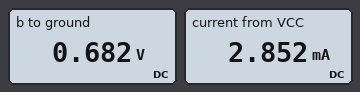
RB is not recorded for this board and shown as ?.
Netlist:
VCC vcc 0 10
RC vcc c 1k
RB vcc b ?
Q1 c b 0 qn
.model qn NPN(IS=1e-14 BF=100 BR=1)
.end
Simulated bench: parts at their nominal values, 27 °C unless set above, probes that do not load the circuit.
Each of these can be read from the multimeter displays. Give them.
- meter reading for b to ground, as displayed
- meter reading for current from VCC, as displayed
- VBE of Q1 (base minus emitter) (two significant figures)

0.682 V
2.852 mA
680 mV
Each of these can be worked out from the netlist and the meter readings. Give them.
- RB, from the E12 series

330 kΩ
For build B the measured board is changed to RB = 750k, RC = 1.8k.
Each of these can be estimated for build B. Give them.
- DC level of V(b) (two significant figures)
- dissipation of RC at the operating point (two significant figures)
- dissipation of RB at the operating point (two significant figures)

660 mV
2.8 mW
120 µW
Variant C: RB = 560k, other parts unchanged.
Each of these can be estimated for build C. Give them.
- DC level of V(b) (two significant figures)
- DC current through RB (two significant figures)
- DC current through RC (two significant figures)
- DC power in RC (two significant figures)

670 mV
17 µA
1.7 mA
2.8 mW
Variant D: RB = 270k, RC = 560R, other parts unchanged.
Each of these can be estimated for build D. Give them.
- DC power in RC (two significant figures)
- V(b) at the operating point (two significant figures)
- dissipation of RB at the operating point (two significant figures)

6.7 mW
690 mV
320 µW
